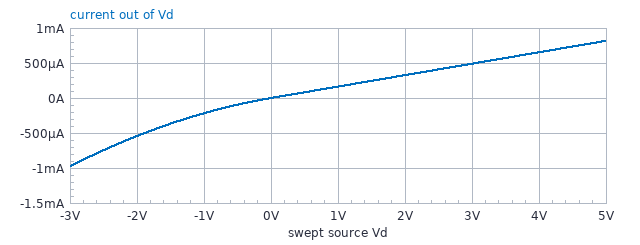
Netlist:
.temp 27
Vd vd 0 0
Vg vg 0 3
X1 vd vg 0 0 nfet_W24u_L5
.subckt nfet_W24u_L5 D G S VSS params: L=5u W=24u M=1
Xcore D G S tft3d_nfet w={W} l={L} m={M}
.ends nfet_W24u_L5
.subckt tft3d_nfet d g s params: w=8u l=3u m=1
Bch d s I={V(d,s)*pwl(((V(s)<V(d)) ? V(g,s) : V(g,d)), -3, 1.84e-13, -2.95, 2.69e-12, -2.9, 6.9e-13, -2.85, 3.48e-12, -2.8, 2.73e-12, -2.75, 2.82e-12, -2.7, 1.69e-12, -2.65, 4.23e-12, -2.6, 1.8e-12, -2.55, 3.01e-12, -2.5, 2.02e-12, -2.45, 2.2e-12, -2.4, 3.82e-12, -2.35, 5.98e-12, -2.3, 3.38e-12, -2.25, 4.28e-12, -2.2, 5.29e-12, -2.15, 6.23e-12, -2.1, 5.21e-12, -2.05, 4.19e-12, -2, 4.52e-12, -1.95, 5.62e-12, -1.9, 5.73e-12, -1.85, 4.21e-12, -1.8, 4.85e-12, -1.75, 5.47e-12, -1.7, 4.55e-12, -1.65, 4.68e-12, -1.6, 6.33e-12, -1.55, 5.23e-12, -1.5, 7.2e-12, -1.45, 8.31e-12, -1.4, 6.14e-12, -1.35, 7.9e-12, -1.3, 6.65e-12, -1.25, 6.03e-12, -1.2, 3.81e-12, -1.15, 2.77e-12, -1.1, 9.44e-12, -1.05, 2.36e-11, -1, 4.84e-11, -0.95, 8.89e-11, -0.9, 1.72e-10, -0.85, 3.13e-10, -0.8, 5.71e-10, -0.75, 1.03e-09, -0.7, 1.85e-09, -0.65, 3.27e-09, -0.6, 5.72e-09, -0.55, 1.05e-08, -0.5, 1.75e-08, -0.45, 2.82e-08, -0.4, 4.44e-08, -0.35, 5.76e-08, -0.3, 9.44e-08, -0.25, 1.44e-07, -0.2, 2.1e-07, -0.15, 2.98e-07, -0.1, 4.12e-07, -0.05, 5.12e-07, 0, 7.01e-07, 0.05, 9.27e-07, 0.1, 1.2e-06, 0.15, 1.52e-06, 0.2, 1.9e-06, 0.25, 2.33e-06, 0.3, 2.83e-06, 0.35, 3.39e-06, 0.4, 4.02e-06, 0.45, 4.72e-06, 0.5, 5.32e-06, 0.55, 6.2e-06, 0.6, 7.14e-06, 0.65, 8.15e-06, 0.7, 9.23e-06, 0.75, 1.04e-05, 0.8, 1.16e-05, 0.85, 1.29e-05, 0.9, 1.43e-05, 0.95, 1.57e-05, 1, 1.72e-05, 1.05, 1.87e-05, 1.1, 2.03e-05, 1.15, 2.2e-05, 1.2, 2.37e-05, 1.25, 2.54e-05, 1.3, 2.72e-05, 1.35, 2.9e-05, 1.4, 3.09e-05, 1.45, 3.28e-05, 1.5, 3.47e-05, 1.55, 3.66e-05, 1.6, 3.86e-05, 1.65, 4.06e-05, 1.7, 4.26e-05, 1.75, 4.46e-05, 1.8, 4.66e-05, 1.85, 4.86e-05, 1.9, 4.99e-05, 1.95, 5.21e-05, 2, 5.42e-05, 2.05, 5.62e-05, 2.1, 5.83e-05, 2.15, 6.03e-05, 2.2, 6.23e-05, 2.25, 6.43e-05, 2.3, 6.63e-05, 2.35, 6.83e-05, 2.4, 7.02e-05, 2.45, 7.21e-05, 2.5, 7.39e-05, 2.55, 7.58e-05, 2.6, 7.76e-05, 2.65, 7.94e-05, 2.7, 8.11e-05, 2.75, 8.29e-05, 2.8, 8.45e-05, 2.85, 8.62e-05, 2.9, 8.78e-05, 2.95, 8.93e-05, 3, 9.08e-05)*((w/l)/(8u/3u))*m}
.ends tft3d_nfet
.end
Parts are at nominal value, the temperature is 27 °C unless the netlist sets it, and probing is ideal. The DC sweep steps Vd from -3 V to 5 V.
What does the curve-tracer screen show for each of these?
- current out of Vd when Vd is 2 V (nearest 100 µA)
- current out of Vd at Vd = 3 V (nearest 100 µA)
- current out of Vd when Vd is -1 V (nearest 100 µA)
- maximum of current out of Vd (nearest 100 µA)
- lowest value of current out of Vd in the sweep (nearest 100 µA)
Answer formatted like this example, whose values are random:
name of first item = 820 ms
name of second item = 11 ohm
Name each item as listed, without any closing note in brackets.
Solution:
current out of Vd when Vd is 2 V = 300 µA
current out of Vd at Vd = 3 V = 500 µA
current out of Vd when Vd is -1 V = -200 µA
maximum of current out of Vd = 800 µA
lowest value of current out of Vd in the sweep = -1.0 mA
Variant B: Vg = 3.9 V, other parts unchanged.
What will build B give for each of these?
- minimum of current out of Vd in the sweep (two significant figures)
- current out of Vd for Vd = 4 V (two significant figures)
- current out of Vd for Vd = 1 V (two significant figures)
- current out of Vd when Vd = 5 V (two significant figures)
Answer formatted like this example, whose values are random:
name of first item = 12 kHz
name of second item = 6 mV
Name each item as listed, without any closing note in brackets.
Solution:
minimum of current out of Vd in the sweep = -1.1 mA
current out of Vd for Vd = 4 V = 850 µA
current out of Vd for Vd = 1 V = 210 µA
current out of Vd when Vd = 5 V = 1.1 mA
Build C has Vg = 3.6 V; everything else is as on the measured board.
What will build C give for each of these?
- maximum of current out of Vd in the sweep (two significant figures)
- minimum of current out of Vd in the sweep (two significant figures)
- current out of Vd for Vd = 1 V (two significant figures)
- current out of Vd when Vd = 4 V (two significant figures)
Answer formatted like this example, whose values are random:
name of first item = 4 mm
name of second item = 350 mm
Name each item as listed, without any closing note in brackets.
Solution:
maximum of current out of Vd in the sweep = 980 µA
minimum of current out of Vd in the sweep = -1.1 mA
current out of Vd for Vd = 1 V = 200 µA
current out of Vd when Vd = 4 V = 780 µA
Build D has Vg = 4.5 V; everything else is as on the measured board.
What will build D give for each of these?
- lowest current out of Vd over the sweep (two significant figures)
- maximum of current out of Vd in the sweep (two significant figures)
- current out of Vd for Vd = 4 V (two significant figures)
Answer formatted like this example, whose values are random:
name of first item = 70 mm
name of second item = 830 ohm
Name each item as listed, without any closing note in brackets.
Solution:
lowest current out of Vd over the sweep = -1.2 mA
maximum of current out of Vd in the sweep = 1.2 mA
current out of Vd for Vd = 4 V = 980 µA
